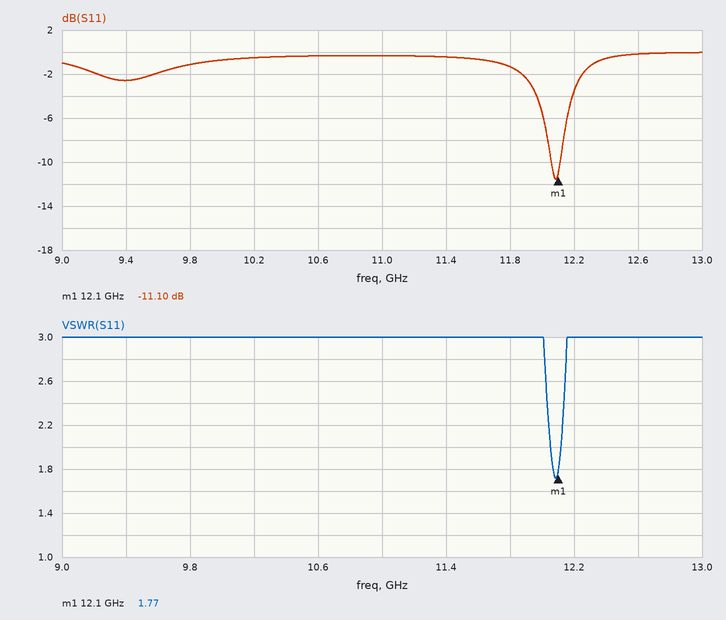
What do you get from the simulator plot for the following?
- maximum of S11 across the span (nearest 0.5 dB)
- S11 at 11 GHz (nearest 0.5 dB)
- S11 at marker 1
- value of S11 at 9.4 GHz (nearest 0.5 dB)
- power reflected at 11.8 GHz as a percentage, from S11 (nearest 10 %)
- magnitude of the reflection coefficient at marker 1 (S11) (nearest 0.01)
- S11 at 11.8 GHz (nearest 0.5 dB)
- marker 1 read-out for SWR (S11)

0.0 dB
-0.5 dB
-11.10 dB
-2.5 dB
70 %
0.28
-1.5 dB
1.77
